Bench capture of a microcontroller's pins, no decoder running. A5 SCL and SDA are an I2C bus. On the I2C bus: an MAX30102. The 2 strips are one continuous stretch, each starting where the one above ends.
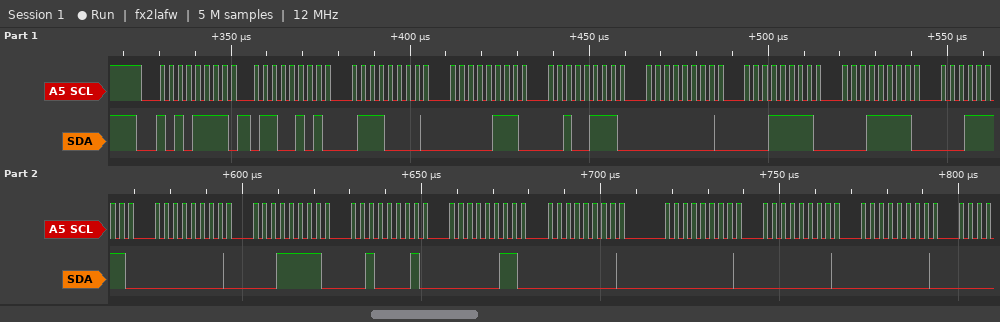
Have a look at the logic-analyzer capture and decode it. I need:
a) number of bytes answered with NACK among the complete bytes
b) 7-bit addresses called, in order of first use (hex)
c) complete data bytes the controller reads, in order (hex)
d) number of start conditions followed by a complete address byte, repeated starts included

0
0x57
65 70 07 27 00 1F 1F 1F 00 1F 21 03 00 00 00 00
1
